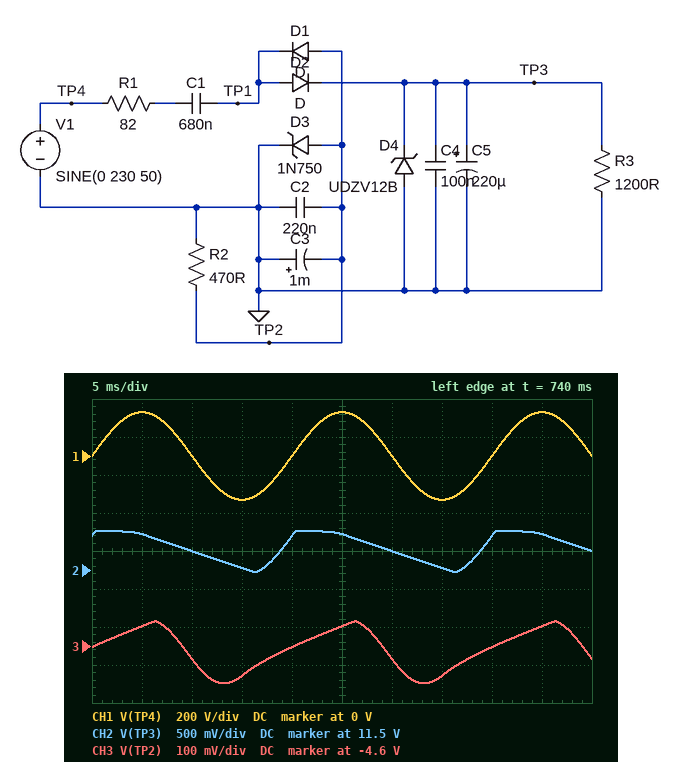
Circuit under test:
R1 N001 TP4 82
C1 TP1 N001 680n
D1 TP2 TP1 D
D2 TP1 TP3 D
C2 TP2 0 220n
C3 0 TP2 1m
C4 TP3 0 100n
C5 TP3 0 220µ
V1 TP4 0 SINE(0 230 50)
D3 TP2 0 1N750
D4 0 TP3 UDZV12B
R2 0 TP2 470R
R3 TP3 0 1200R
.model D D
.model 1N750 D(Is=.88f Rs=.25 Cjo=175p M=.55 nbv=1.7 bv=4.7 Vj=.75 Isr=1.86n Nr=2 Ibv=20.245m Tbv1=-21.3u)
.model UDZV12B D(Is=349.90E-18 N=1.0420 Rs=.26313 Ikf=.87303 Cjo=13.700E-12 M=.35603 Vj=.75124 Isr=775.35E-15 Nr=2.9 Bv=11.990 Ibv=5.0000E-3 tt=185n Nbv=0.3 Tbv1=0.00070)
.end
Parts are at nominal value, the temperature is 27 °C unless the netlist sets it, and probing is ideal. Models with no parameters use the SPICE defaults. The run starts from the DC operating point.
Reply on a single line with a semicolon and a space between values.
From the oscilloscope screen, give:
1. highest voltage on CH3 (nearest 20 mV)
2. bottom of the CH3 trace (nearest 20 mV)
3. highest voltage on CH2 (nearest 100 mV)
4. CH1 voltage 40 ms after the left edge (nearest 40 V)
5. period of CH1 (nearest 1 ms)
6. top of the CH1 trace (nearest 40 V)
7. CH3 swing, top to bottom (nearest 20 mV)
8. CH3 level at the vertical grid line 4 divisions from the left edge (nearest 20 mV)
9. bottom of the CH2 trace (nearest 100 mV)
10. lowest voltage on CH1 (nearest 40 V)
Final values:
-4.54 V; -4.70 V; 12.0 V; 0 V; 20 ms; 240 V; 160 mV; -4.60 V; 11.5 V; -240 V
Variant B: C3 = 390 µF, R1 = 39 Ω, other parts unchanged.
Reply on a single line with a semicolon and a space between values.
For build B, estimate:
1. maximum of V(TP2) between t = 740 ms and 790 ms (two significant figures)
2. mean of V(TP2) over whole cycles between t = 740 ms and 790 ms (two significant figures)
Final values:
-4.4 V; -4.5 V
